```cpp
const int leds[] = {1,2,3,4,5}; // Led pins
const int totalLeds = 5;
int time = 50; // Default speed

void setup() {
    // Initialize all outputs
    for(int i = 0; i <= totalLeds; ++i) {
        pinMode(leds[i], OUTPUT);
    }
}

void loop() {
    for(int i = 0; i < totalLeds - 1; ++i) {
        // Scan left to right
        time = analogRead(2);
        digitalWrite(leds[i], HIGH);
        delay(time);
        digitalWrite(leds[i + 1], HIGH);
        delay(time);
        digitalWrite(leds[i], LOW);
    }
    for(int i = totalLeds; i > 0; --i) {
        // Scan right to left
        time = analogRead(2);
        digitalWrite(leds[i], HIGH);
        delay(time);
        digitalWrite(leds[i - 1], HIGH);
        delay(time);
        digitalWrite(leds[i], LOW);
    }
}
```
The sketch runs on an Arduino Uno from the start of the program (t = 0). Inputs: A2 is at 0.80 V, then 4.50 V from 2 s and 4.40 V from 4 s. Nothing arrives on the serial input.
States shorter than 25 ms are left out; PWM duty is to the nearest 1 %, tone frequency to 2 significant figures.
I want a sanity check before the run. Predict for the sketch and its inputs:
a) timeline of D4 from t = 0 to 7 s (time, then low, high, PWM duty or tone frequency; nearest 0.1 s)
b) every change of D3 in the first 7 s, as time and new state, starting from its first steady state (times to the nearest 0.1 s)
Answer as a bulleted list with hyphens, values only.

- 0 s low; 0.8 s high; 1.3 s low; 1.8 s high; 2.3 s low
- 0 s low; 0.5 s high; 1 s low; 2.1 s high; 4.1 s low
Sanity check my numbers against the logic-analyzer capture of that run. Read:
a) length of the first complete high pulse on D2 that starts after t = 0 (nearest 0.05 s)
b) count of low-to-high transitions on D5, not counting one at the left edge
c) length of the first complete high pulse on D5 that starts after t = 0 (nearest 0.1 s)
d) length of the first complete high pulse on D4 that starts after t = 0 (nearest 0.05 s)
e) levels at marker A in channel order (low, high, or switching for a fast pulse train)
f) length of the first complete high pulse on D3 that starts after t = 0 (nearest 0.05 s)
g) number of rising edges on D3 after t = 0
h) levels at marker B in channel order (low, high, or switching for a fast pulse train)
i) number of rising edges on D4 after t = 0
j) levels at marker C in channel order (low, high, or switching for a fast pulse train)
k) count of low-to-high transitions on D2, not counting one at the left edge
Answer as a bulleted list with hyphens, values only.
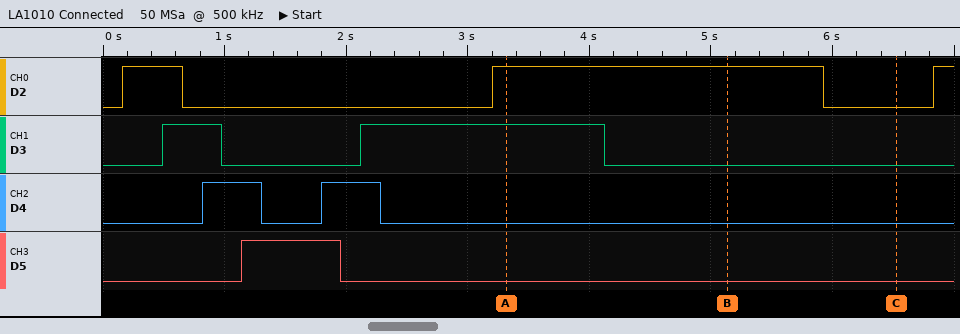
- 0.50 s
- 1
- 0.8 s
- 0.50 s
- D2 high, D3 high, D4 low, D5 low
- 0.50 s
- 2
- D2 high, D3 low, D4 low, D5 low
- 2
- D2 low, D3 low, D4 low, D5 low
- 3
